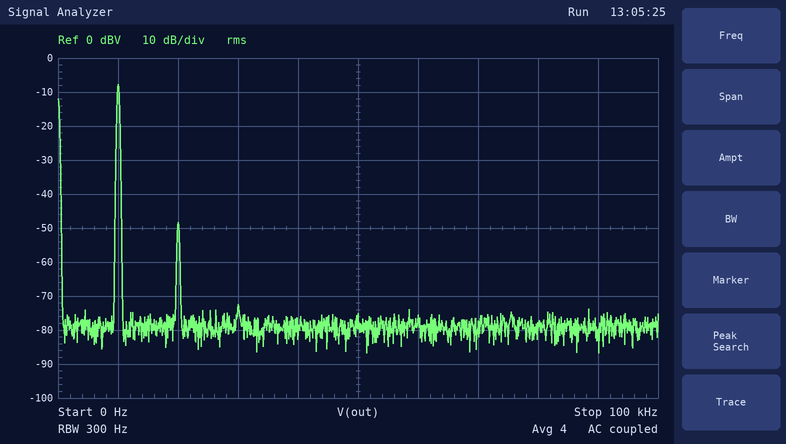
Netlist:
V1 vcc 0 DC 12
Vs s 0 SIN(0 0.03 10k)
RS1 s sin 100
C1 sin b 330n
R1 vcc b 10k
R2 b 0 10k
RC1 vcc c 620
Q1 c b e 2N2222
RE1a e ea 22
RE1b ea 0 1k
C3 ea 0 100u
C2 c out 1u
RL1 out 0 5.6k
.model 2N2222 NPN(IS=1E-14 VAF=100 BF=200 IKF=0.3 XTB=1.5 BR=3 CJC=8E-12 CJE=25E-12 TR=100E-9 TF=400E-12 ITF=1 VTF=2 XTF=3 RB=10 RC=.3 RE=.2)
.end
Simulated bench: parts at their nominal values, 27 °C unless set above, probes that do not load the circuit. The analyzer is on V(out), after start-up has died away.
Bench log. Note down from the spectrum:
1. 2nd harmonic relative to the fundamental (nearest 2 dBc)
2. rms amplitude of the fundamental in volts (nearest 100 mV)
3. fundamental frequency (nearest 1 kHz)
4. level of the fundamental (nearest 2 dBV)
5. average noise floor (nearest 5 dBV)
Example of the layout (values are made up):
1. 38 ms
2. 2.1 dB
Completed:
1. -40 dBc
2. 400 mV
3. 10 kHz
4. -8 dBV
5. -80 dBV
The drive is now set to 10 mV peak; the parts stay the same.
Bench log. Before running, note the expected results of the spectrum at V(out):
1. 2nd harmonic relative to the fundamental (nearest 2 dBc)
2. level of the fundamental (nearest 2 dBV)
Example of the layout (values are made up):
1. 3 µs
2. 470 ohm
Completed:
1. -50 dBc
2. -18 dBV
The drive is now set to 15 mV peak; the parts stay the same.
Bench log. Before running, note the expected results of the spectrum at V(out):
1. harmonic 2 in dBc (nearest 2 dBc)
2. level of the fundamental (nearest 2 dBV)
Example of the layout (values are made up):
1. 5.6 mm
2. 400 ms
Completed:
1. -46 dBc
2. -14 dBV
